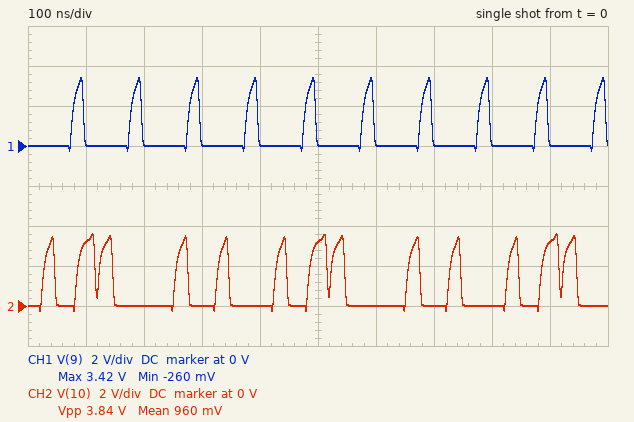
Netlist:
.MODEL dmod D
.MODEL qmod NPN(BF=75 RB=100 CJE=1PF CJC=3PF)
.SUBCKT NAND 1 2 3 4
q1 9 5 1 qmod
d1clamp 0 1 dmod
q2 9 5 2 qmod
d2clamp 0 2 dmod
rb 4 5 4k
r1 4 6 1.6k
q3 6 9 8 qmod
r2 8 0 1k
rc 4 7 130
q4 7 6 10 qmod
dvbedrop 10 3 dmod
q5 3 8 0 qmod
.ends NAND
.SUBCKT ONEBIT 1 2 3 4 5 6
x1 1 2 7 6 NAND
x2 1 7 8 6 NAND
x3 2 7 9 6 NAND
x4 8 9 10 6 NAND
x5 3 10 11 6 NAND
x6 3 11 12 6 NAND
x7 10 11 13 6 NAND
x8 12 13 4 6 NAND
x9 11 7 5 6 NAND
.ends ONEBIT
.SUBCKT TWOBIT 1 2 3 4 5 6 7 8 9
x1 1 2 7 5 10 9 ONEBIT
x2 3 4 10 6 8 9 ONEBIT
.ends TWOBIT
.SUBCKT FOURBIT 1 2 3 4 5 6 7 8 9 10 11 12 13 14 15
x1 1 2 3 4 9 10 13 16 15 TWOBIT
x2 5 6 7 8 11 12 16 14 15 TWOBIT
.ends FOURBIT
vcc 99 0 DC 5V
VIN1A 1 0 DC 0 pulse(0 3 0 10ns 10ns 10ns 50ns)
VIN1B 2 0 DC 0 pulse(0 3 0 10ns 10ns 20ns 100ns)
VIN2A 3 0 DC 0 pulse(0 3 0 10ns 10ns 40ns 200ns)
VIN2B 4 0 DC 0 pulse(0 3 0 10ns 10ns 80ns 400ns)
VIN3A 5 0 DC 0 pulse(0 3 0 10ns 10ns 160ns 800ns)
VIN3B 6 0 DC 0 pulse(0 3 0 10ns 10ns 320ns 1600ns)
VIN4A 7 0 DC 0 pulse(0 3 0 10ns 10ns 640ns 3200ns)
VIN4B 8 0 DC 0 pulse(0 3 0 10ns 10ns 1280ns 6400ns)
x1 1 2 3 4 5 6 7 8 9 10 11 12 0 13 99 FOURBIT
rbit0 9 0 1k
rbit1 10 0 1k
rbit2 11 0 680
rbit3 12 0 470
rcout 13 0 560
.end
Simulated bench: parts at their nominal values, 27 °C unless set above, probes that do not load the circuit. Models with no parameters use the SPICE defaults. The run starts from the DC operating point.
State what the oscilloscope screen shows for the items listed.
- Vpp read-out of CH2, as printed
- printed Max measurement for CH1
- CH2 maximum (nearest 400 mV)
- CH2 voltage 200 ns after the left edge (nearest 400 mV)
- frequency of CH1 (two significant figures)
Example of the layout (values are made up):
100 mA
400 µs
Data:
3.84 V
3.42 V
3.6 V
0 V
10 MHz
